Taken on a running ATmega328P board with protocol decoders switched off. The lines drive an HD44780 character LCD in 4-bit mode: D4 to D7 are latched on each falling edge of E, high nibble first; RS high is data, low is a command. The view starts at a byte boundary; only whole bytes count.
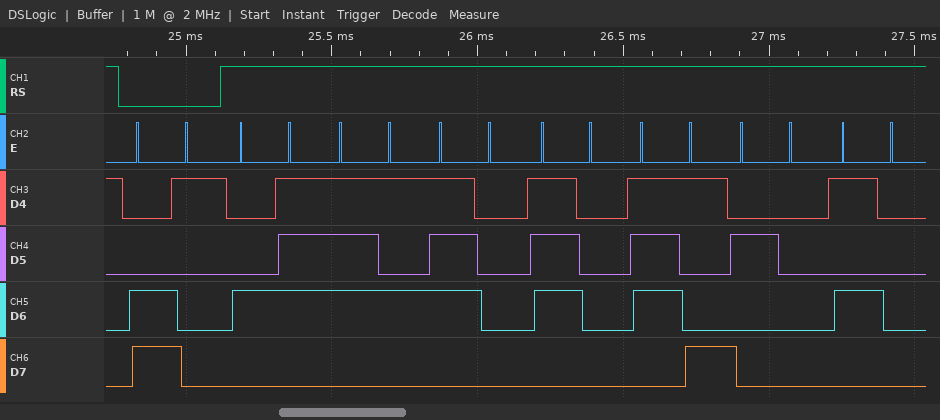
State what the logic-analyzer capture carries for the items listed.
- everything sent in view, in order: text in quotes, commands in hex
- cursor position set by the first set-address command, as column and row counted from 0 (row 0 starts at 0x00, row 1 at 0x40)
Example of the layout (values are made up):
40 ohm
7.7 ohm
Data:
0xC1 "Guppy P"
column 1, row 1
